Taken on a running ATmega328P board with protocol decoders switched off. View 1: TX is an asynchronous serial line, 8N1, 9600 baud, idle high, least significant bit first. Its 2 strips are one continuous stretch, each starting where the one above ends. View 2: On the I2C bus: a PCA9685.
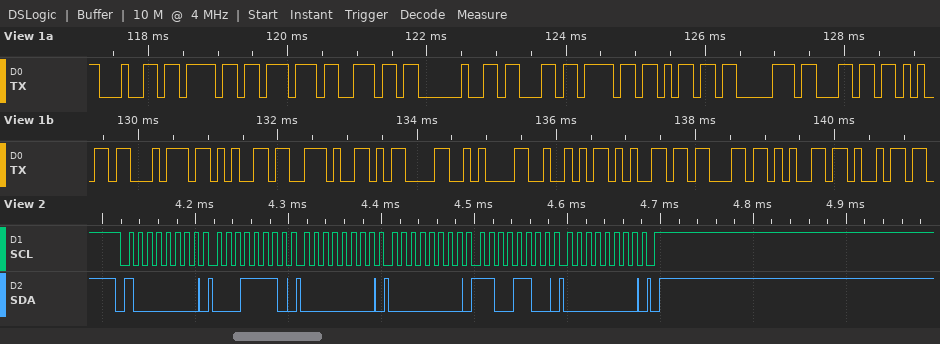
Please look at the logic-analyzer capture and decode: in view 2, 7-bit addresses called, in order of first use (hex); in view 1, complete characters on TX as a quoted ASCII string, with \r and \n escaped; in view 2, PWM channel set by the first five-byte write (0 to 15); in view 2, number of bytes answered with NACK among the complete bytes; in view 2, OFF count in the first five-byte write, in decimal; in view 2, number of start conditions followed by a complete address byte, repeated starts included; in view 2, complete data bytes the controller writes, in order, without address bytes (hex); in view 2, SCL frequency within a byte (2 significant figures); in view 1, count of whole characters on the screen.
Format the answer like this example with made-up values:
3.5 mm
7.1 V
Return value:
0x40
"down complete.\r\nRecei"
6
0
204
1
1E 00 00 CC 00
100 kHz
21
